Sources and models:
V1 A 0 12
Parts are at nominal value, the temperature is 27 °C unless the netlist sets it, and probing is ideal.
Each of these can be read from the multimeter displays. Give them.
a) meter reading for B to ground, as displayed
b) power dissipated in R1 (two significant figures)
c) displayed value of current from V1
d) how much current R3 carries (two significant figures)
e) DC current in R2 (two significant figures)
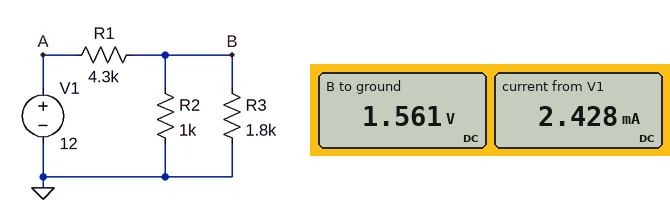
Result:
1.561 V
25 mW
2.428 mA
870 µA
1.6 mA
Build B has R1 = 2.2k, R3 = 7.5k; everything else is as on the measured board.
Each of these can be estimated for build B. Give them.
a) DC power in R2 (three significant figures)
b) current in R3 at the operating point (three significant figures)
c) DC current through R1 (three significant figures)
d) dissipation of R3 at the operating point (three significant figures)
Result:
11.8 mW
458 µA
3.89 mA
1.57 mW
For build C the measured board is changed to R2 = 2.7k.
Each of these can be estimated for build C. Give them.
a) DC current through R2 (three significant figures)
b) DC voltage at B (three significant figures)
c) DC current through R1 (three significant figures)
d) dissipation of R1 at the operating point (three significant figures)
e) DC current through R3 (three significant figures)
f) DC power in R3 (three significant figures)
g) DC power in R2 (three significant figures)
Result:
892 µA
2.41 V
2.23 mA
21.4 mW
1.34 mA
3.22 mW
2.15 mW
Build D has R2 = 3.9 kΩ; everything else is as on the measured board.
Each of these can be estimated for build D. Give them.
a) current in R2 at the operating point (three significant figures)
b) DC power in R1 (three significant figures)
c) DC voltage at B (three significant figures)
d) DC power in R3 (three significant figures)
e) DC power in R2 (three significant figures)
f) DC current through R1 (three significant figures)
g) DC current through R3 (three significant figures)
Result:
685 µA
20.2 mW
2.67 V
3.97 mW
1.83 mW
2.17 mA
1.48 mA
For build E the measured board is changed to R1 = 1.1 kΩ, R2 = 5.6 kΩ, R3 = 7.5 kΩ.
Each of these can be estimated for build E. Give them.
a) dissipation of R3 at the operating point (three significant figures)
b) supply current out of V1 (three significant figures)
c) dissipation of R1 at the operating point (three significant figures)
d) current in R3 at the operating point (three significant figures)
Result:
10.6 mW
2.79 mA
8.54 mW
1.19 mA
